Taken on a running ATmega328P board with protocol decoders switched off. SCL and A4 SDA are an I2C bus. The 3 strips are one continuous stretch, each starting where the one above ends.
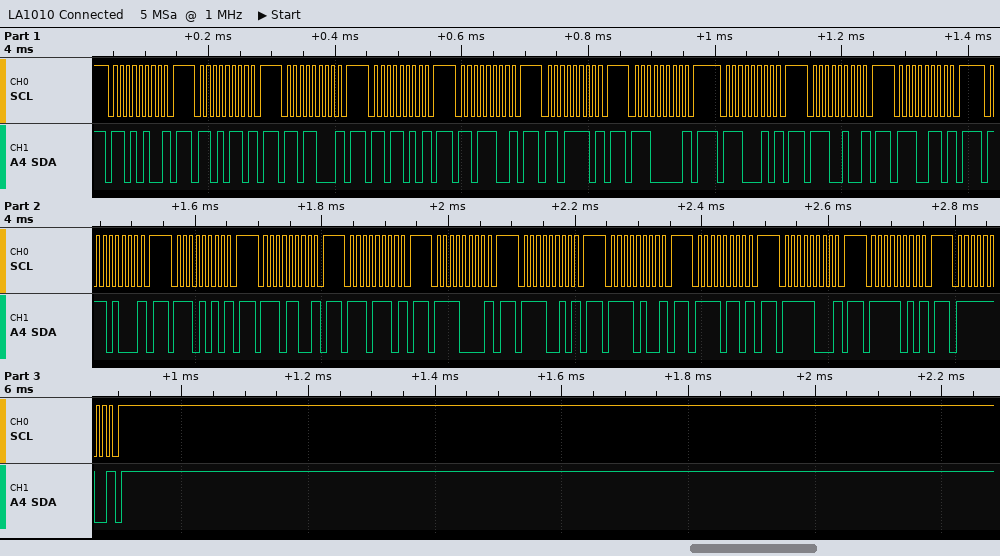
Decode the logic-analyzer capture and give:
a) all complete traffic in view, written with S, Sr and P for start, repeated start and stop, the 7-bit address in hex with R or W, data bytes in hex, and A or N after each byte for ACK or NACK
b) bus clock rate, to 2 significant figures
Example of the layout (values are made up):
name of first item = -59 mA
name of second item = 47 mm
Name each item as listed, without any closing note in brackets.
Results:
all complete traffic in view, written with S, Sr and P for start, repeated start and stop, the 7-bit address in hex with R or W, data bytes in hex, and A or N after each byte for ACK or NACK = S 6AW N P S 6BW N P S 6CW N P S 6DW N P S 6EW N P S 6FW N P S 70W N P S 71W N P S 72W N P S 73W N P S 74W N P S 75W N P S 76W N P S 77W N P S 78W N P S 79W N P S 7AW N P S 7BW N P S 7CW N P S 7DW N P S 7EW N P
bus clock rate, to 2 significant figures = 100 kHz
